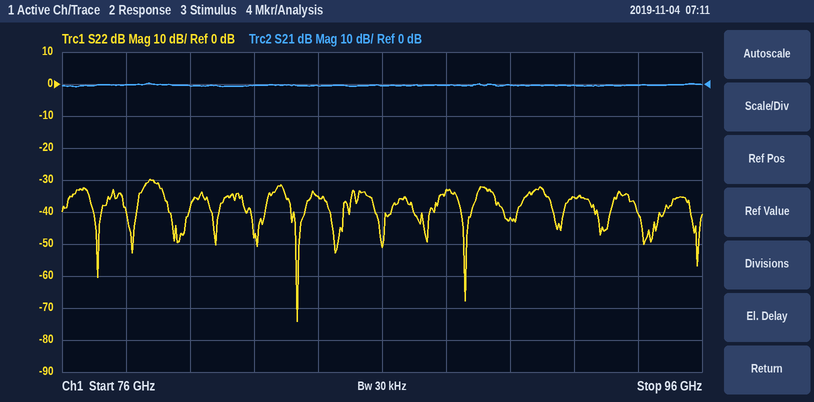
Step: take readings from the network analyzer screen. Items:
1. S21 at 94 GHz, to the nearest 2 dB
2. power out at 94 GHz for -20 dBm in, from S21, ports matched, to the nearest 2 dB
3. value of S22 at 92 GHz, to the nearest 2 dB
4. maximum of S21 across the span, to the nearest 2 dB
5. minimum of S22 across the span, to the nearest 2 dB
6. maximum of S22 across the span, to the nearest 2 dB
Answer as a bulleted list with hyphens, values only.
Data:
- 0 dB
- -20 dBm
- -36 dB
- 0 dB
- -74 dB
- -30 dB
